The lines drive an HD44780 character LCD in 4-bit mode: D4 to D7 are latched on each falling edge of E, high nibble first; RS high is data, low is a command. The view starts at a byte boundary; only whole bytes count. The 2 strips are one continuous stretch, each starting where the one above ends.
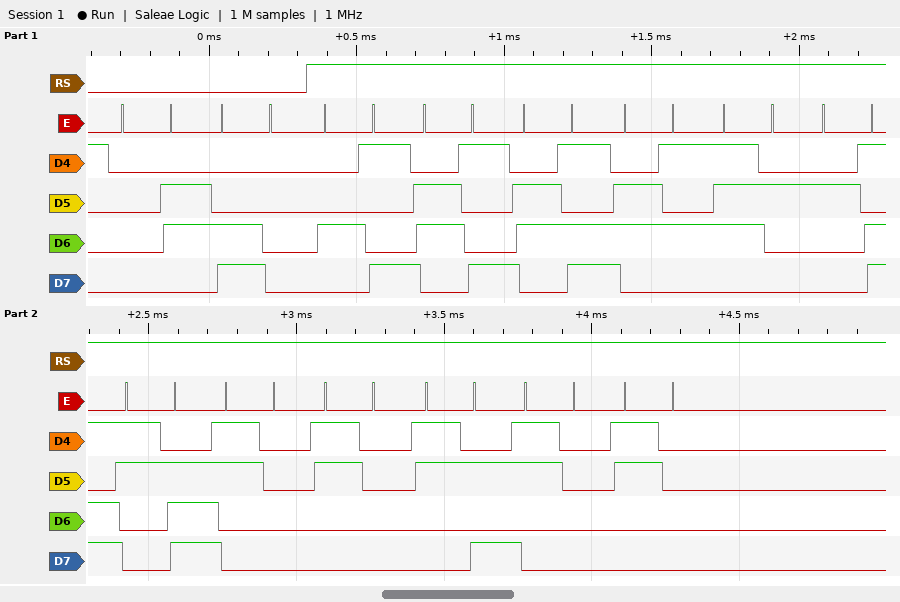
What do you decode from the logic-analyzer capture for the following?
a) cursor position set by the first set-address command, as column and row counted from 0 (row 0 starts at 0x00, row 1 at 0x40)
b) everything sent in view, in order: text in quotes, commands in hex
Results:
column 0, row 1
0x06 0xC0 "Iimer->00:00"
